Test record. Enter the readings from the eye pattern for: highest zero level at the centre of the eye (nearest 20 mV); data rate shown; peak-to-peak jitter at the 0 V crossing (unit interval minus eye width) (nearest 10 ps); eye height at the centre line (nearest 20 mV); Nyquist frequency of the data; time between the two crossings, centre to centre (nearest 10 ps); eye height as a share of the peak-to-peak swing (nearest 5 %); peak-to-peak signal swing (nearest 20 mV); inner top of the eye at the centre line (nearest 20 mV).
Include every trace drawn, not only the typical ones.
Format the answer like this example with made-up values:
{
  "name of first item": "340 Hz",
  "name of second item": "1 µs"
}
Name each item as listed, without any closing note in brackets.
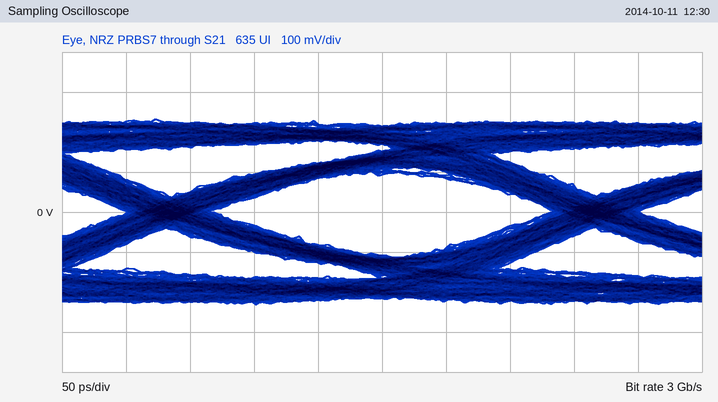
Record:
{
  "highest zero level at the centre of the eye": "-100 mV",
  "data rate shown": "3 Gb/s",
  "peak-to-peak jitter at the 0 V crossing (unit interval minus eye width)": "70 ps",
  "eye height at the centre line": "200 mV",
  "Nyquist frequency of the data": "1.5 GHz",
  "time between the two crossings, centre to centre": "330 ps",
  "eye height as a share of the peak-to-peak swing": "45 %",
  "peak-to-peak signal swing": "460 mV",
  "inner top of the eye at the centre line": "100 mV"
}
